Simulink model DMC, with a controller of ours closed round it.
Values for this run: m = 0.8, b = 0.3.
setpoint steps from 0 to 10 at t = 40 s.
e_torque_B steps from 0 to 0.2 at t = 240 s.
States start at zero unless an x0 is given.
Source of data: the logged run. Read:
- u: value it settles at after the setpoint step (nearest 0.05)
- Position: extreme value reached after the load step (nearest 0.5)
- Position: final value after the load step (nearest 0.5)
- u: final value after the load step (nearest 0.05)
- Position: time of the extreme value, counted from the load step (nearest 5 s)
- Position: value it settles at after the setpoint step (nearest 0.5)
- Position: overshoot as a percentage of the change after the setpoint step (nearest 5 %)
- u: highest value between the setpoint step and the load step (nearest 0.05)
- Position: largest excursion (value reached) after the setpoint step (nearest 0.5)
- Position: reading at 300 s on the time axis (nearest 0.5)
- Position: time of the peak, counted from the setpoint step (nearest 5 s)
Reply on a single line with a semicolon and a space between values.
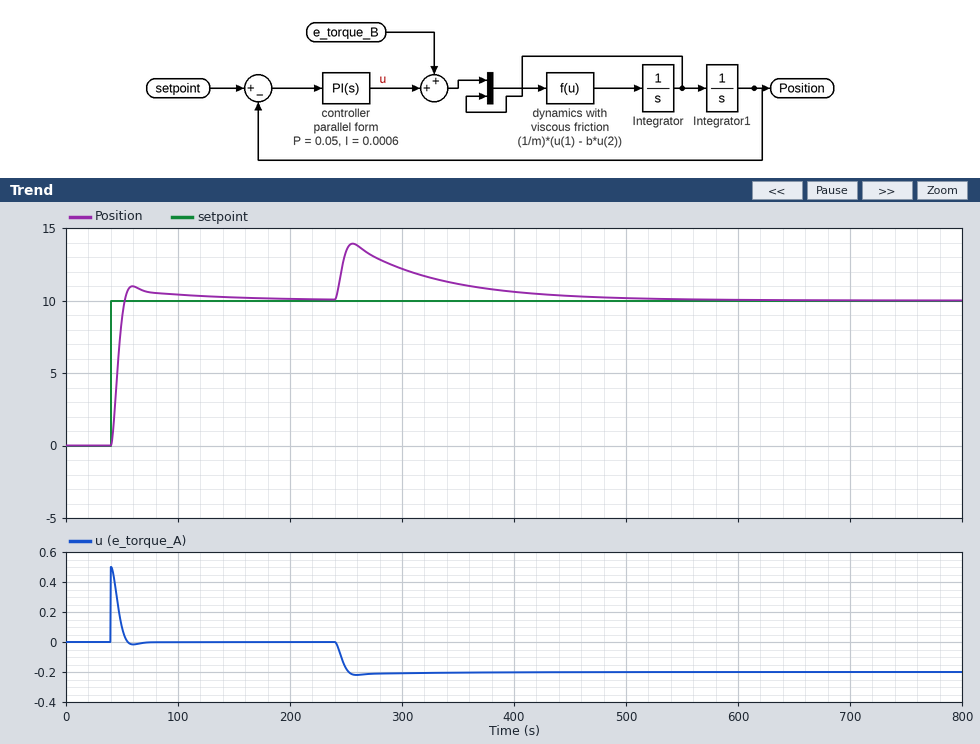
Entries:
0.00; 14.0; 10.0; -0.20; 15 s; 10.0; 10 %; 0.50; 11.0; 12.0; 20 s
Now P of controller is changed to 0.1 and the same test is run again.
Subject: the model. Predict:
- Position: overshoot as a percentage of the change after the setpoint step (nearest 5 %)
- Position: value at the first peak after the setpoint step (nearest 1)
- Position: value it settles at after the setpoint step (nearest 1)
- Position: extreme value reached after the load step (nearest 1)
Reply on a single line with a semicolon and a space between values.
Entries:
15 %; 12; 10; 12
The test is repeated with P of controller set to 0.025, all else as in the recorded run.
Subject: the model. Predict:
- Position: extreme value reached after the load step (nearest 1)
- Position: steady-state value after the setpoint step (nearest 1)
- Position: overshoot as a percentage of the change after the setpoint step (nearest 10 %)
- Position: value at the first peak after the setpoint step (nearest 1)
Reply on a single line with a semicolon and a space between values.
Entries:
16; 10; 20 %; 12
